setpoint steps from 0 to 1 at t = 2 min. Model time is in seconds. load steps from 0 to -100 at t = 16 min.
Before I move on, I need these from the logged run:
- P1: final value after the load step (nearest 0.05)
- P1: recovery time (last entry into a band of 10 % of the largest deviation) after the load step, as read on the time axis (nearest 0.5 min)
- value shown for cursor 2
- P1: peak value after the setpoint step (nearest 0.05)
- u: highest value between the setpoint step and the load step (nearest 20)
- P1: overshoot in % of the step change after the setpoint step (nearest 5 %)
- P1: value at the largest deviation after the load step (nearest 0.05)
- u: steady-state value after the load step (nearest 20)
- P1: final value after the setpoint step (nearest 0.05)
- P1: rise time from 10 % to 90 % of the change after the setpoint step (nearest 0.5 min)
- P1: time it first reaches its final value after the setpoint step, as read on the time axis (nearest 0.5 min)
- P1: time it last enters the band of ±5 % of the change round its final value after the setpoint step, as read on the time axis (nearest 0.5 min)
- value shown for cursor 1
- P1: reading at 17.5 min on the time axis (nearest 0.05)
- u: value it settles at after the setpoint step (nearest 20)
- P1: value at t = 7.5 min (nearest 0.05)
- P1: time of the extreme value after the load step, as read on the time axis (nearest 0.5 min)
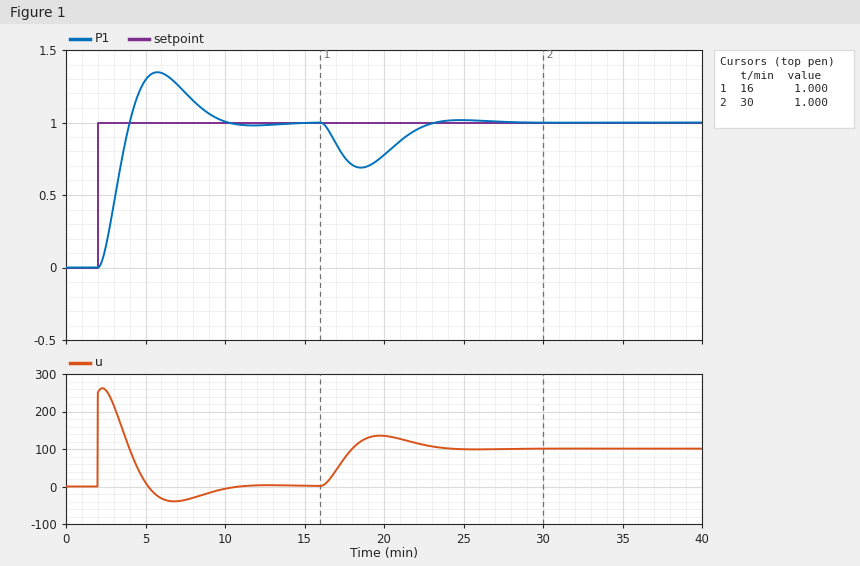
1.00
22.5 min
1.000
1.35
260
35 %
0.70
100
1.00
1.5 min
4.0 min
9.0 min
1.000
0.75
0
1.20
18.5 min
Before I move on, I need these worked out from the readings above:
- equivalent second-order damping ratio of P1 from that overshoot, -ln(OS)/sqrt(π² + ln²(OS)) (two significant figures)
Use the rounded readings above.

0.32
